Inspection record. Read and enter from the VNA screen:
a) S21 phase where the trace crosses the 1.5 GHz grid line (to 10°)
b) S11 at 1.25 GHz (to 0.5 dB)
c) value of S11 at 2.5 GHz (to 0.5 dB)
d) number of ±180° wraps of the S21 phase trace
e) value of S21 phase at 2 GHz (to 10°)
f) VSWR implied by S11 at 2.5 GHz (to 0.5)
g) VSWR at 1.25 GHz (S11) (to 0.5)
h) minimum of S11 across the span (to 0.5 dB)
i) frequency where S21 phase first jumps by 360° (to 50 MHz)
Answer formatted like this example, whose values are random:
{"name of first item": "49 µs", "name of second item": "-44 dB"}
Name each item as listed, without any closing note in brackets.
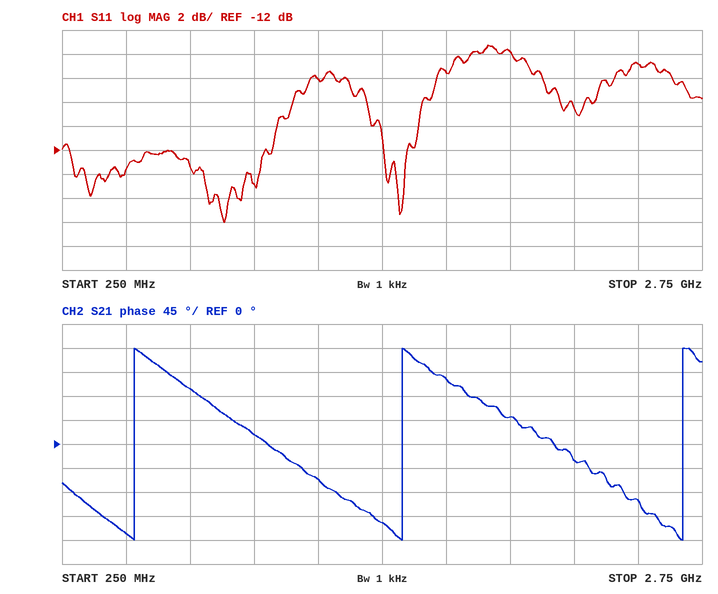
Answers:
{"S21 phase where the trace crosses the 1.5 GHz grid line": "-150°", "S11 at 1.25 GHz": "-6.0 dB", "value of S11 at 2.5 GHz": "-5.0 dB", "number of ±180° wraps of the S21 phase trace": "3", "value of S21 phase at 2 GHz": "50°", "VSWR implied by S11 at 2.5 GHz": "3.5", "VSWR at 1.25 GHz (S11)": "3.0", "minimum of S11 across the span": "-18.0 dB", "frequency where S21 phase first jumps by 360°": "550 MHz"}
